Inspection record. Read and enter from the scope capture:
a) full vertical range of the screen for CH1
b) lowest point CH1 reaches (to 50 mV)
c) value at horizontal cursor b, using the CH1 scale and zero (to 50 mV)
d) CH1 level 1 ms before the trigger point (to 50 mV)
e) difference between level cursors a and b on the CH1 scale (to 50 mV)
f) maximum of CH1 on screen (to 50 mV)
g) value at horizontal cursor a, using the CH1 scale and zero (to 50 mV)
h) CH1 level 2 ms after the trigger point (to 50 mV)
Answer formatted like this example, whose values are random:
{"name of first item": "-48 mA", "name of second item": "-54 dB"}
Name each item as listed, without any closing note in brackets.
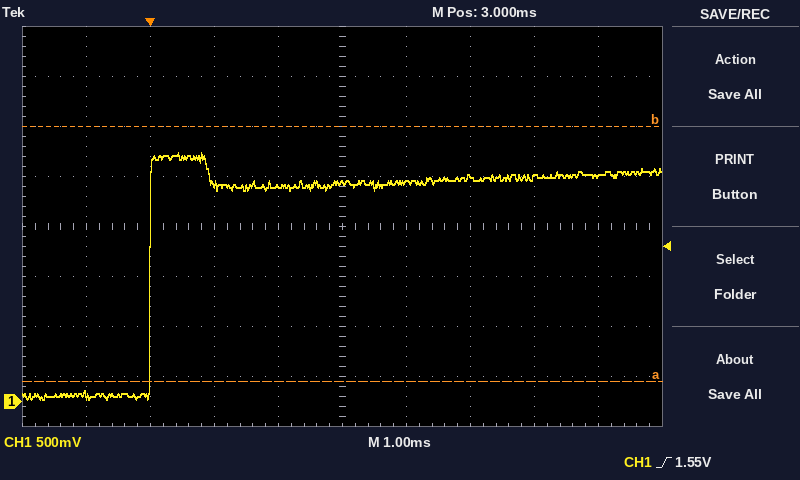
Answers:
{"full vertical range of the screen for CH1": "4 V", "lowest point CH1 reaches": "0 mV", "value at horizontal cursor b, using the CH1 scale and zero": "2.75 V", "CH1 level 1 ms before the trigger point": "50 mV", "difference between level cursors a and b on the CH1 scale": "2.55 V", "maximum of CH1 on screen": "2.50 V", "value at horizontal cursor a, using the CH1 scale and zero": "200 mV", "CH1 level 2 ms after the trigger point": "2.15 V"}
